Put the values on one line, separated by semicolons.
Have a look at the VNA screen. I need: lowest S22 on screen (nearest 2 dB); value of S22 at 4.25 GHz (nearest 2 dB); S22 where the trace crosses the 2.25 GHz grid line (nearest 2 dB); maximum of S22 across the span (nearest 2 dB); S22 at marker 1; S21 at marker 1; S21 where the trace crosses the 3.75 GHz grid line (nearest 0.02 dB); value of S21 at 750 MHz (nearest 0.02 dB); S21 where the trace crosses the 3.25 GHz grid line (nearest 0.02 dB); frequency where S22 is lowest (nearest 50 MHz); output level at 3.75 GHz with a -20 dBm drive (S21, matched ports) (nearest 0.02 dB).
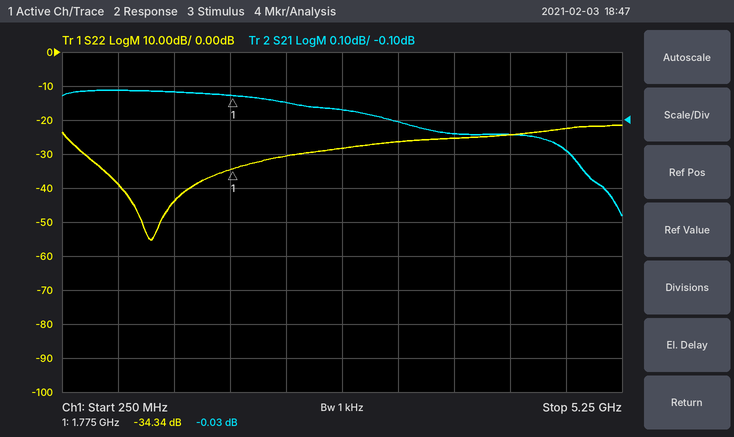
-56 dB; -24 dB; -30 dB; -22 dB; -34.34 dB; -0.03 dB; -0.14 dB; -0.02 dB; -0.10 dB; 1.05 GHz; -20.14 dBm
